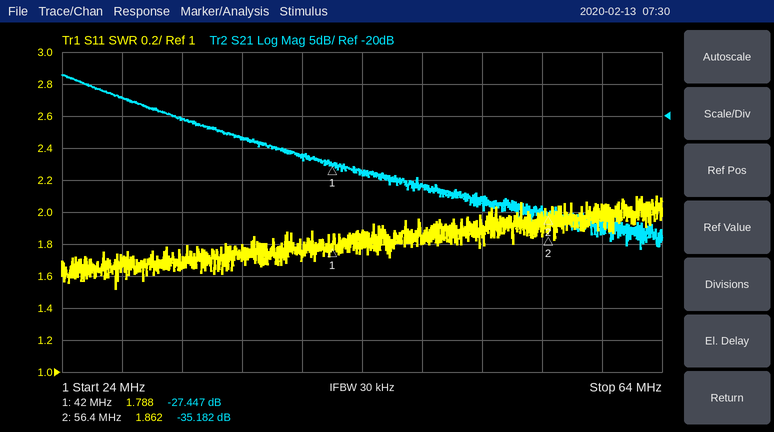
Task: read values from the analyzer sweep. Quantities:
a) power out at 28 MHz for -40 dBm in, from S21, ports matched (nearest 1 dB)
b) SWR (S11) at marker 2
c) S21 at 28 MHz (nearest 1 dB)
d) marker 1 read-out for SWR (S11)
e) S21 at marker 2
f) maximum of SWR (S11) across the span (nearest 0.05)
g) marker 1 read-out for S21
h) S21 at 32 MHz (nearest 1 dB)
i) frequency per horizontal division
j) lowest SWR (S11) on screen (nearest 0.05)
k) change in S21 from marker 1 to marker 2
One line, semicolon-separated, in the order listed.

-57 dBm; 1.862; -17 dB; 1.788; -35.182 dB; 2.10; -27.447 dB; -20 dB; 4 MHz; 1.50; -7.735 dB
